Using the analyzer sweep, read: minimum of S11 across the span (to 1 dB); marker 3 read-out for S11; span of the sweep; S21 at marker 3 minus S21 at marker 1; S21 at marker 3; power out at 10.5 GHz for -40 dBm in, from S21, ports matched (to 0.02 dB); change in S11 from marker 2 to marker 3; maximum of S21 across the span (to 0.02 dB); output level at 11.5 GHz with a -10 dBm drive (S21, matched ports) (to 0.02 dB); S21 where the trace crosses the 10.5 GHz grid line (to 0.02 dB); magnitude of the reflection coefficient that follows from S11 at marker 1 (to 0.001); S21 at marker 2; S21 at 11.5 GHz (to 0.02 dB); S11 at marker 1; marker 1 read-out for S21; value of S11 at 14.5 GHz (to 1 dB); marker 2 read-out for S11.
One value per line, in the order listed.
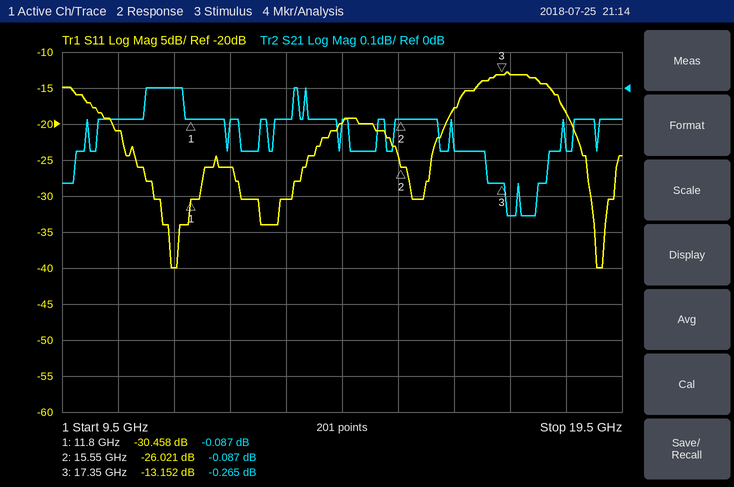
-40 dB
-13.152 dB
10 GHz
-0.178 dB
-0.265 dB
-40.08 dBm
12.869 dB
0.00 dB
-10.00 dBm
-0.08 dB
0.030
-0.087 dB
0.00 dB
-30.458 dB
-0.087 dB
-20 dB
-26.021 dB
